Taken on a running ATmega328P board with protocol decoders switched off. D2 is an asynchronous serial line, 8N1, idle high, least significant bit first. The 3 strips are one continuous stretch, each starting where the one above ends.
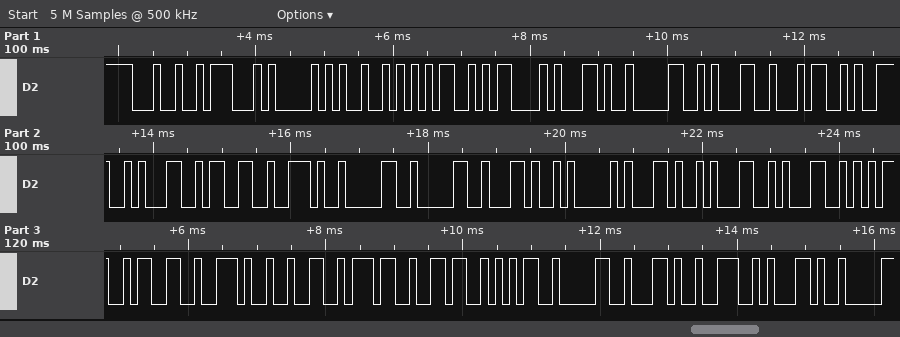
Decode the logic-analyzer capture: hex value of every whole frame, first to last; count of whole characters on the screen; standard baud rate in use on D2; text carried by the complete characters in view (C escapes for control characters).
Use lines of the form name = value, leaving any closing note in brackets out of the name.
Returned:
hex value of every whole frame, first to last = 24 47 50 52 4D 43 2C 30 31 34 39 31 33 2E 30 30 2C 41 2C 31 31 35 33 2E 32 37 36 35 30 2C 4E 2C
count of whole characters on the screen = 32
standard baud rate in use on D2 = 9600 baud
text carried by the complete characters in view = "$GPRMC,014913.00,A,1153.27650,N,"
